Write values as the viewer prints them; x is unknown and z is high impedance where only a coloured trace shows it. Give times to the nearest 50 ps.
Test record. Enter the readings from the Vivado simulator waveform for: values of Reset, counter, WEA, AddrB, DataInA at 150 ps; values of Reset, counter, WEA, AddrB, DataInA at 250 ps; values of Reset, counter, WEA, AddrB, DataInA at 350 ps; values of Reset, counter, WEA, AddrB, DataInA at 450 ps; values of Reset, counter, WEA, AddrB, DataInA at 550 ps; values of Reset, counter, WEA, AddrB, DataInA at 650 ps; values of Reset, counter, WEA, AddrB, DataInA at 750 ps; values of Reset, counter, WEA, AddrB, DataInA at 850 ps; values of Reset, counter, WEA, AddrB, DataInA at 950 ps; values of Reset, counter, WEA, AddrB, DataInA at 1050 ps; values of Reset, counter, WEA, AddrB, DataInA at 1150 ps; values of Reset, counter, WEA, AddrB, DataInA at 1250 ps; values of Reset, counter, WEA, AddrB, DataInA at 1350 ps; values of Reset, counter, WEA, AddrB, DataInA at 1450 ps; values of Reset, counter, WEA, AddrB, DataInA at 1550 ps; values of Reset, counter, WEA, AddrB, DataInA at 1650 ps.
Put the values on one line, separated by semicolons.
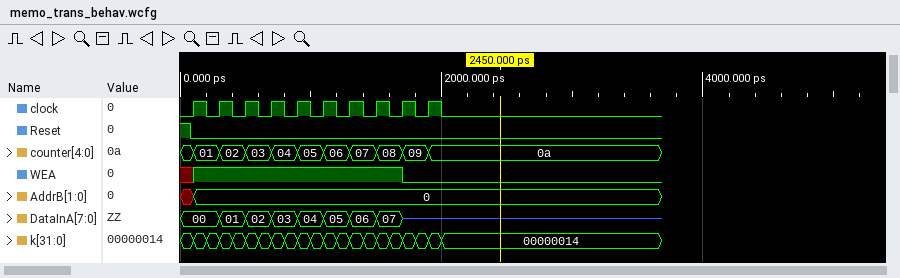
Reset=0, counter=01, WEA=1, AddrB=0, DataInA=00; Reset=0, counter=01, WEA=1, AddrB=0, DataInA=00; Reset=0, counter=02, WEA=1, AddrB=0, DataInA=01; Reset=0, counter=02, WEA=1, AddrB=0, DataInA=01; Reset=0, counter=03, WEA=1, AddrB=0, DataInA=02; Reset=0, counter=03, WEA=1, AddrB=0, DataInA=02; Reset=0, counter=04, WEA=1, AddrB=0, DataInA=03; Reset=0, counter=04, WEA=1, AddrB=0, DataInA=03; Reset=0, counter=05, WEA=1, AddrB=0, DataInA=04; Reset=0, counter=05, WEA=1, AddrB=0, DataInA=04; Reset=0, counter=06, WEA=1, AddrB=0, DataInA=05; Reset=0, counter=06, WEA=1, AddrB=0, DataInA=05; Reset=0, counter=07, WEA=1, AddrB=0, DataInA=06; Reset=0, counter=07, WEA=1, AddrB=0, DataInA=06; Reset=0, counter=08, WEA=1, AddrB=0, DataInA=07; Reset=0, counter=08, WEA=1, AddrB=0, DataInA=07
